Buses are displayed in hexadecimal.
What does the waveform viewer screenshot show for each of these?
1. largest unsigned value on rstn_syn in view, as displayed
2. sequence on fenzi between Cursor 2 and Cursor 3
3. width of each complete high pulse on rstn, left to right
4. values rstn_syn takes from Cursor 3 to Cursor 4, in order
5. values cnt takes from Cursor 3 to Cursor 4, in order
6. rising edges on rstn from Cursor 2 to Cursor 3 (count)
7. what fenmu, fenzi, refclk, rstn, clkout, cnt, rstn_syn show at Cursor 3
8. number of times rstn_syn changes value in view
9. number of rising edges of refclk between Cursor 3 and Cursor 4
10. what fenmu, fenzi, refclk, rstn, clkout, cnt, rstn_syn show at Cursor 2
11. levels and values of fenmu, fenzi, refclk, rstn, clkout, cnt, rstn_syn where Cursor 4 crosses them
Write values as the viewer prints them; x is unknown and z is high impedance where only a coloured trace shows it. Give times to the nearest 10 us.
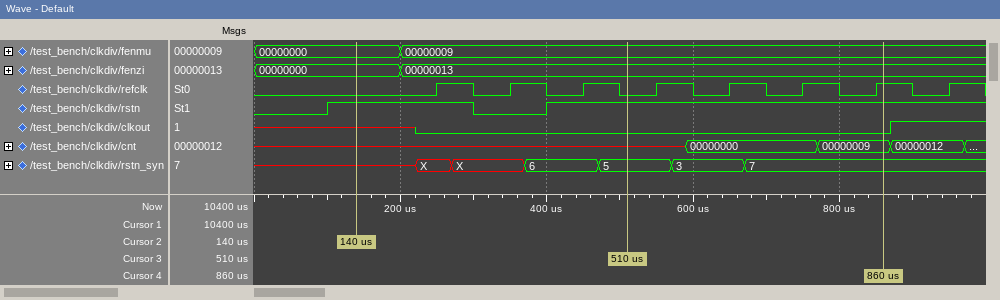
7
00000000, 00000013
200 us
5, 3, 7
x, 00000000, 00000009
1
fenmu=00000009, fenzi=00000013, refclk=0, rstn=1, clkout=0, cnt=x, rstn_syn=5
6
4
fenmu=00000000, fenzi=00000000, refclk=0, rstn=1, clkout=x, cnt=x, rstn_syn=x
fenmu=00000009, fenzi=00000013, refclk=1, rstn=1, clkout=0, cnt=00000009, rstn_syn=7
